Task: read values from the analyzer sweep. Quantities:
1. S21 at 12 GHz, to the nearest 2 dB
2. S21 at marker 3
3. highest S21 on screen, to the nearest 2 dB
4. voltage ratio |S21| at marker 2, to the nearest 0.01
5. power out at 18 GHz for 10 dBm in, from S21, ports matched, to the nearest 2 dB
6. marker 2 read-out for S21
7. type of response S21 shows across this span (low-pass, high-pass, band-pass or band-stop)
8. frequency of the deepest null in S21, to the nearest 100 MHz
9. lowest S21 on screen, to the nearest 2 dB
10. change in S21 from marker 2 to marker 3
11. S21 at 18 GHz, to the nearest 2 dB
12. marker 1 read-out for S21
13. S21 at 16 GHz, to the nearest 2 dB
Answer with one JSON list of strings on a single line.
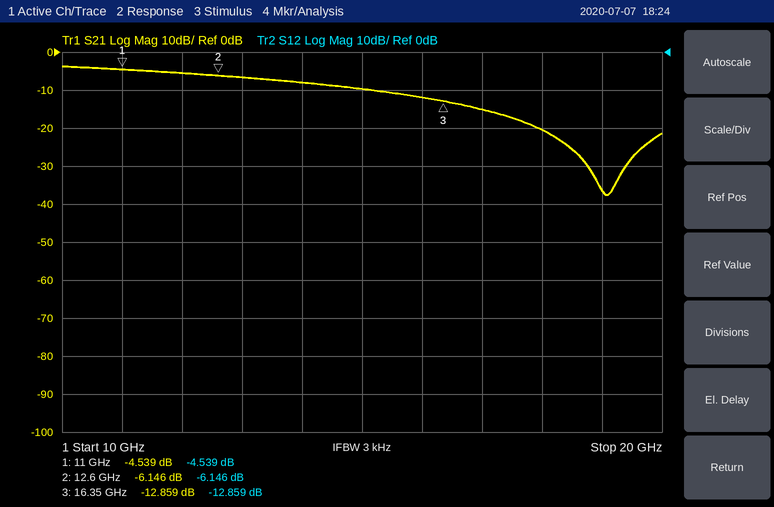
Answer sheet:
["-6 dB", "-12.859 dB", "-4 dB", "0.49", "-10 dBm", "-6.146 dB", "low-pass", "19.1 GHz", "-38 dB", "-6.713 dB", "-20 dB", "-4.539 dB", "-12 dB"]
